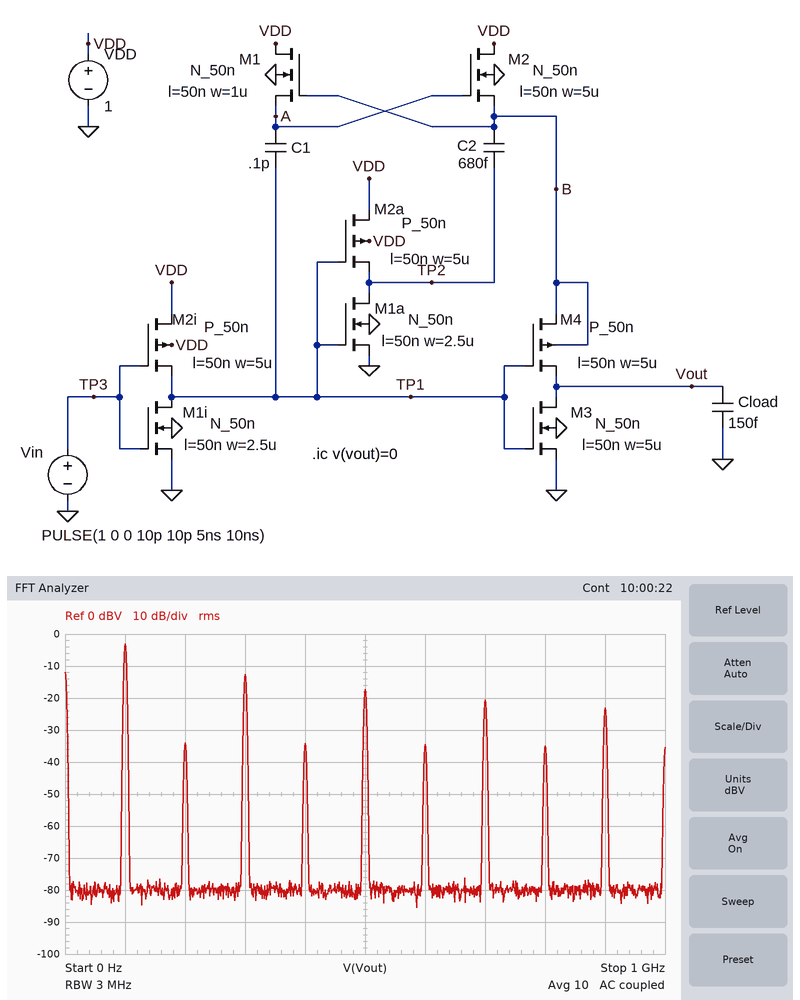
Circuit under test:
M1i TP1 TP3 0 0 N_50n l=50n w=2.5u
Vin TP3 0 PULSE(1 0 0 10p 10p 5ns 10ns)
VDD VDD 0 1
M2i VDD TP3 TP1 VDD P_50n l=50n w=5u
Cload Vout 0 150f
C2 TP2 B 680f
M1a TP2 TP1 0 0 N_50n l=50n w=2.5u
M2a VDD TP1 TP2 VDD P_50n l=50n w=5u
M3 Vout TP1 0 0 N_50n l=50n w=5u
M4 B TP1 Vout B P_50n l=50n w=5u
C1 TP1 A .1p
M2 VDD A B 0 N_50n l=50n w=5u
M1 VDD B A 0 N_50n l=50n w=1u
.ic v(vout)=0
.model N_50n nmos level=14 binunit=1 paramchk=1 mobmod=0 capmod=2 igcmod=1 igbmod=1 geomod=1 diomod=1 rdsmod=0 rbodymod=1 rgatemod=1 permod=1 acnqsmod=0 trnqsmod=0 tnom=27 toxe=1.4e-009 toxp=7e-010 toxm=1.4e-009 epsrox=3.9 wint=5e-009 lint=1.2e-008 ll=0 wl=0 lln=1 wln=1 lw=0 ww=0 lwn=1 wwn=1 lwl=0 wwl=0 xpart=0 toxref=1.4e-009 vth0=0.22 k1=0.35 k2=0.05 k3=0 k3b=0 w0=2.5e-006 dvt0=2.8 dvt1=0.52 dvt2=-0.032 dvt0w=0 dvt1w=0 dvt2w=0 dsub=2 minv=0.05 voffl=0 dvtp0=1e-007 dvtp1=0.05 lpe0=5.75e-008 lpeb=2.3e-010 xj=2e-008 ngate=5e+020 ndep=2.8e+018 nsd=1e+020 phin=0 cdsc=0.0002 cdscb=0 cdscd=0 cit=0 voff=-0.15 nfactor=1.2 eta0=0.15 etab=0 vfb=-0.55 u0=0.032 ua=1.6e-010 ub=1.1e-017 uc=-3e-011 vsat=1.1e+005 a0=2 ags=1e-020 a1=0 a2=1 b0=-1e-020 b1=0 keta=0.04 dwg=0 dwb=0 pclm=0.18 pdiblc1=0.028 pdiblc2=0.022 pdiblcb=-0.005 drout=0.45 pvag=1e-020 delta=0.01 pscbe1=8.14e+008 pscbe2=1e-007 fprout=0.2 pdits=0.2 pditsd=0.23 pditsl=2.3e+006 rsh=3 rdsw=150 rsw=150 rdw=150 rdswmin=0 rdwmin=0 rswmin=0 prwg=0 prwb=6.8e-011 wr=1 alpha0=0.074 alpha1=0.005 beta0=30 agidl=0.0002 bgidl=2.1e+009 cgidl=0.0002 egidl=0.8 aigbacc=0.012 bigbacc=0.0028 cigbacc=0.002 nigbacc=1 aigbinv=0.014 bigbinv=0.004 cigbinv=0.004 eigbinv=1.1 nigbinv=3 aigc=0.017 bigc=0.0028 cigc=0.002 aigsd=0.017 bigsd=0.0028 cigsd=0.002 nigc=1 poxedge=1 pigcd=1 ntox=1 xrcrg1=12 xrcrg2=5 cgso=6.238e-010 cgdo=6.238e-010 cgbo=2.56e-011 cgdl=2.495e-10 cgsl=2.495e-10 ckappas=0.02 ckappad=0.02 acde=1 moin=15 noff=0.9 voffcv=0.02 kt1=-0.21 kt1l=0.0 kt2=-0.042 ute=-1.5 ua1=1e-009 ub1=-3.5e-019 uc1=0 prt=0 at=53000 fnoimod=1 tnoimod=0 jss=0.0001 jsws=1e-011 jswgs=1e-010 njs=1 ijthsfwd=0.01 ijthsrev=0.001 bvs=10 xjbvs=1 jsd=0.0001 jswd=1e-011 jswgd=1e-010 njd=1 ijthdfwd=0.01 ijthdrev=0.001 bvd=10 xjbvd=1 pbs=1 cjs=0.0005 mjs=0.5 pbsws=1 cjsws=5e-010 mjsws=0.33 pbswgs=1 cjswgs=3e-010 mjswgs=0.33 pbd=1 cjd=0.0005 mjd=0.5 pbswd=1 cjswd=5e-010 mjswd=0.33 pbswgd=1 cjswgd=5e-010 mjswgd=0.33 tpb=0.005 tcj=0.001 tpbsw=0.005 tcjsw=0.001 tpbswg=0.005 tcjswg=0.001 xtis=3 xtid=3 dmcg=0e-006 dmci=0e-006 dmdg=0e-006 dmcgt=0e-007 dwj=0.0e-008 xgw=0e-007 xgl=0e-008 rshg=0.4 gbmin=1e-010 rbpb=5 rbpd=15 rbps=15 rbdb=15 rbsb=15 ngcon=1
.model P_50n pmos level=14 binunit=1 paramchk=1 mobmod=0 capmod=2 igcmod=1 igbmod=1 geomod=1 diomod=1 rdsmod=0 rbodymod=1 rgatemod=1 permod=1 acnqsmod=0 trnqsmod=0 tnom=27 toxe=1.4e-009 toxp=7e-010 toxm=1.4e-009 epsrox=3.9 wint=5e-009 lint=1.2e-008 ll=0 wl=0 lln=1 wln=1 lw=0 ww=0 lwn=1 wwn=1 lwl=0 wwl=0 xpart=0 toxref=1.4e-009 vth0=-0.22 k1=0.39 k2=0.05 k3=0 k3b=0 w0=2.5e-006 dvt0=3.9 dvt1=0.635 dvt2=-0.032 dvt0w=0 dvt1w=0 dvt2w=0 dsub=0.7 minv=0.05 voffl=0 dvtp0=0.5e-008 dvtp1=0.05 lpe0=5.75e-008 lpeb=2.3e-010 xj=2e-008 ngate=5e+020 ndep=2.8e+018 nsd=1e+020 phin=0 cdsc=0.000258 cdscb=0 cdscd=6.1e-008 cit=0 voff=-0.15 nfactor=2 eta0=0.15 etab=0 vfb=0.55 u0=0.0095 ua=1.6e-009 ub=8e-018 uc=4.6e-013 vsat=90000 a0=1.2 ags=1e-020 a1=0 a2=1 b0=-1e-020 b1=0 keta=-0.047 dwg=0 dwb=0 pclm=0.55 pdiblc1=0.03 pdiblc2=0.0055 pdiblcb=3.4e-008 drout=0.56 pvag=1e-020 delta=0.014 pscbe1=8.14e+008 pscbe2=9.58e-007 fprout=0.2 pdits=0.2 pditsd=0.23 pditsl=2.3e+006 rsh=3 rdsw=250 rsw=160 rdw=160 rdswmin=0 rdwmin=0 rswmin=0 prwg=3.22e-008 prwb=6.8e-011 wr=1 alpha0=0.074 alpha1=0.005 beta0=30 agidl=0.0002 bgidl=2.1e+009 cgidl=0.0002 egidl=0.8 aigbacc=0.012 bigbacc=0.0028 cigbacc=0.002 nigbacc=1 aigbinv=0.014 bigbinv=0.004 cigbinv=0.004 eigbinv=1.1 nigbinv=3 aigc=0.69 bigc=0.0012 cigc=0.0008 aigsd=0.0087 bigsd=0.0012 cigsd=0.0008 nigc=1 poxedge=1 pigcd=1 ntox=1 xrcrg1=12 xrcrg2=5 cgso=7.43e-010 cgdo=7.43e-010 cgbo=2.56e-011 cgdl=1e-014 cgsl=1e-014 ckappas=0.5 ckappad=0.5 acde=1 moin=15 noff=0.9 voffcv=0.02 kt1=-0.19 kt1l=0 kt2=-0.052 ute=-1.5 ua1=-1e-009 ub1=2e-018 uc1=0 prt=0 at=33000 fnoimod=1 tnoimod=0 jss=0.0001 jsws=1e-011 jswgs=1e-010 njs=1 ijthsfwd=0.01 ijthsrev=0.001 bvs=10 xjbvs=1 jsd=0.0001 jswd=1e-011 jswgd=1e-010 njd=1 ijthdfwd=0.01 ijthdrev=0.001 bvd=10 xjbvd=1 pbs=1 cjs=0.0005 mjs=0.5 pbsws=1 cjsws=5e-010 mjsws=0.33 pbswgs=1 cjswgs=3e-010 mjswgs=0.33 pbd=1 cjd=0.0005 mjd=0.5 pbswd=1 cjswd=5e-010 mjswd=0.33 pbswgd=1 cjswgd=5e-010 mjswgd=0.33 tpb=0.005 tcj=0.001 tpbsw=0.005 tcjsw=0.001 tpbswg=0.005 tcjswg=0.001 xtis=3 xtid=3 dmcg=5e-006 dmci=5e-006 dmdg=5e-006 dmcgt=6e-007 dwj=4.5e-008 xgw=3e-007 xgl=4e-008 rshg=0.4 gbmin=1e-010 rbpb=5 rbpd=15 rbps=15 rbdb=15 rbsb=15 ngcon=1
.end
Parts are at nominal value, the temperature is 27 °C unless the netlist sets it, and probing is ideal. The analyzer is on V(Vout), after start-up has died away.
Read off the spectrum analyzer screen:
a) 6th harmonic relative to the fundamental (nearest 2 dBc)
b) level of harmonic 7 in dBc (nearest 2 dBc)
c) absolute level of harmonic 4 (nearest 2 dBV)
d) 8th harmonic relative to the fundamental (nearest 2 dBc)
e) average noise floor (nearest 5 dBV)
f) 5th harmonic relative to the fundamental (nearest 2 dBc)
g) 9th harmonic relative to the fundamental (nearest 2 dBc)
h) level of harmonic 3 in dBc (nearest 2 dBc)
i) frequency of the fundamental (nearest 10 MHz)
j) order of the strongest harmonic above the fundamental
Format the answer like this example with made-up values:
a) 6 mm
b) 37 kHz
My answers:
a) -32 dBc
b) -18 dBc
c) -34 dBV
d) -32 dBc
e) -80 dBV
f) -14 dBc
g) -20 dBc
h) -10 dBc
i) 100 MHz
j) 3
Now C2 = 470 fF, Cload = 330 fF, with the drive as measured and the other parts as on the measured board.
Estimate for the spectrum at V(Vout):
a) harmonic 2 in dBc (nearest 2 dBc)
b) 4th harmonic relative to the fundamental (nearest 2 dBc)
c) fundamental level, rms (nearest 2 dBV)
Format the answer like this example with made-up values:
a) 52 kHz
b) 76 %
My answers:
a) -28 dBc
b) -28 dBc
c) -6 dBV
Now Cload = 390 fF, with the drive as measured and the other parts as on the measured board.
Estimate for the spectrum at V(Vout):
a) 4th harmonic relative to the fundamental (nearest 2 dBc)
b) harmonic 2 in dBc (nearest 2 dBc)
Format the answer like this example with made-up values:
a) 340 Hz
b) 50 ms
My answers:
a) -28 dBc
b) -26 dBc
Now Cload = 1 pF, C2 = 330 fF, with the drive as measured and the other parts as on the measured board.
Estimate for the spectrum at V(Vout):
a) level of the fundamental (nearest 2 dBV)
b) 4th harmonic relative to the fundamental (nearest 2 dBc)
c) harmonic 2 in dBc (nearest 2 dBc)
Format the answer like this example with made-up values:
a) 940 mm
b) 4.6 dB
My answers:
a) -14 dBV
b) -28 dBc
c) -26 dBc
